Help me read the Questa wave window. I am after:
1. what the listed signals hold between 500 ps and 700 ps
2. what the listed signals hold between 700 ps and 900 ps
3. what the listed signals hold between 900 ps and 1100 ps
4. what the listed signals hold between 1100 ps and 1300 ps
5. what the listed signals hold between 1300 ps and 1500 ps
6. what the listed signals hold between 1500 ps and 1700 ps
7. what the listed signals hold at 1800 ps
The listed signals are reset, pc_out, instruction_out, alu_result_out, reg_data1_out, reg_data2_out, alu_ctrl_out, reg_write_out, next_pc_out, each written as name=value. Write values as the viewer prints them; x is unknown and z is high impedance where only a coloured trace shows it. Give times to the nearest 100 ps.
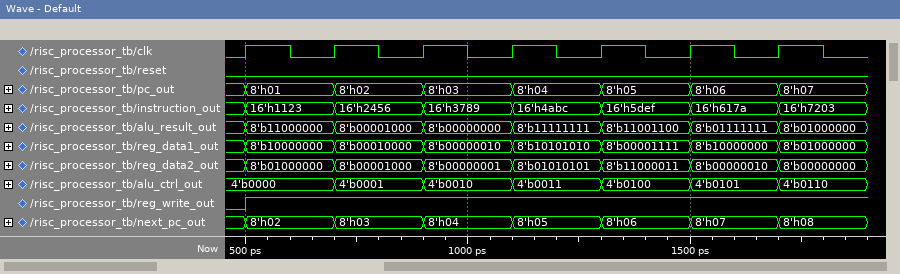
reset=0, pc_out=8'h01, instruction_out=16'h1123, alu_result_out=8'b11000000, reg_data1_out=8'b10000000, reg_data2_out=8'b01000000, alu_ctrl_out=4'b0000, reg_write_out=1, next_pc_out=8'h02
reset=0, pc_out=8'h02, instruction_out=16'h2456, alu_result_out=8'b00001000, reg_data1_out=8'b00010000, reg_data2_out=8'b00001000, alu_ctrl_out=4'b0001, reg_write_out=1, next_pc_out=8'h03
reset=0, pc_out=8'h03, instruction_out=16'h3789, alu_result_out=8'b00000000, reg_data1_out=8'b00000010, reg_data2_out=8'b00000001, alu_ctrl_out=4'b0010, reg_write_out=1, next_pc_out=8'h04
reset=0, pc_out=8'h04, instruction_out=16'h4abc, alu_result_out=8'b11111111, reg_data1_out=8'b10101010, reg_data2_out=8'b01010101, alu_ctrl_out=4'b0011, reg_write_out=1, next_pc_out=8'h05
reset=0, pc_out=8'h05, instruction_out=16'h5def, alu_result_out=8'b11001100, reg_data1_out=8'b00001111, reg_data2_out=8'b11000011, alu_ctrl_out=4'b0100, reg_write_out=1, next_pc_out=8'h06
reset=0, pc_out=8'h06, instruction_out=16'h617a, alu_result_out=8'b01111111, reg_data1_out=8'b10000000, reg_data2_out=8'b00000010, alu_ctrl_out=4'b0101, reg_write_out=1, next_pc_out=8'h07
reset=0, pc_out=8'h07, instruction_out=16'h7203, alu_result_out=8'b01000000, reg_data1_out=8'b01000000, reg_data2_out=8'b00000000, alu_ctrl_out=4'b0110, reg_write_out=1, next_pc_out=8'h08
